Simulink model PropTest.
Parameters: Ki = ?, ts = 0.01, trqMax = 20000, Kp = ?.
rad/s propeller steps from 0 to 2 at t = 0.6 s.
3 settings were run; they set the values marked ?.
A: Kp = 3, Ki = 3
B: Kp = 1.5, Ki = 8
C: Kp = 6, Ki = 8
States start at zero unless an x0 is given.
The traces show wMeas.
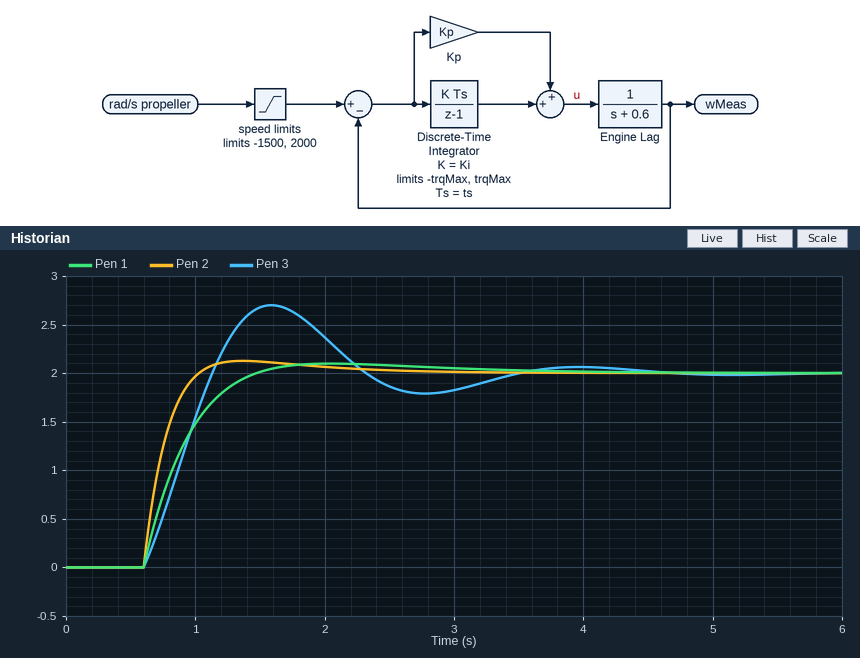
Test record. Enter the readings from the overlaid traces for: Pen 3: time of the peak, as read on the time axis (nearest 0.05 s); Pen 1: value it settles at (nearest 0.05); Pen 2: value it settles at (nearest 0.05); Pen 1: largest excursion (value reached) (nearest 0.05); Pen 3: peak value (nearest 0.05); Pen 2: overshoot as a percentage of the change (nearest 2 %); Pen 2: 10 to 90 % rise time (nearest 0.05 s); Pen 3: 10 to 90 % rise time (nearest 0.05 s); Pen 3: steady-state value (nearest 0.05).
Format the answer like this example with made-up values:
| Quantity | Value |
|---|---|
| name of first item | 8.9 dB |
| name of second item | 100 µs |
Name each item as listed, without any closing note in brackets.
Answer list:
| Quantity | Value |
|---|---|
| Pen 3: time of the peak, as read on the time axis | 1.60 s |
| Pen 1: value it settles at | 2.00 |
| Pen 2: value it settles at | 2.00 |
| Pen 1: largest excursion (value reached) | 2.10 |
| Pen 3: peak value | 2.70 |
| Pen 2: overshoot as a percentage of the change | 6 % |
| Pen 2: 10 to 90 % rise time | 0.30 s |
| Pen 3: 10 to 90 % rise time | 0.40 s |
| Pen 3: steady-state value | 2.00 |
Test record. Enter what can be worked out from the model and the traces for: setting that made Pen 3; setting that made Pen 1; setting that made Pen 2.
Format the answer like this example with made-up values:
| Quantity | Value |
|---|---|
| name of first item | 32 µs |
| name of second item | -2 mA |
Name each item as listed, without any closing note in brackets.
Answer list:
| Quantity | Value |
|---|---|
| setting that made Pen 3 | B |
| setting that made Pen 1 | A |
| setting that made Pen 2 | C |
